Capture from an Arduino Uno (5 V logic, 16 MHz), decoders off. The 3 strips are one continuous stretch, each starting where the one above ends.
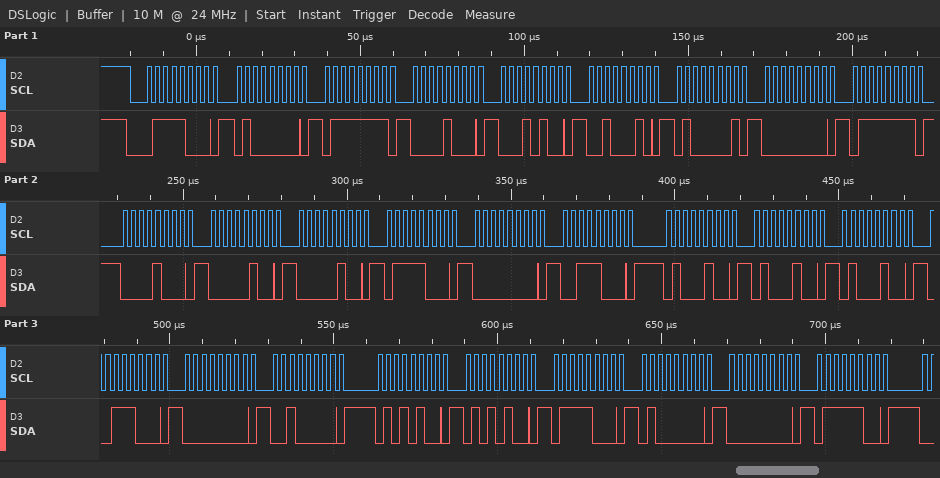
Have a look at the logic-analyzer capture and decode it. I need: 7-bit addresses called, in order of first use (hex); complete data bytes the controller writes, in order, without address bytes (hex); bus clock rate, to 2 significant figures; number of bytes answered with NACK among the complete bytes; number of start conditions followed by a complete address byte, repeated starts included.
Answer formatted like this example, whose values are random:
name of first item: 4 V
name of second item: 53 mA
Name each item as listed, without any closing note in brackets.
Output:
7-bit addresses called, in order of first use: 0x3C
complete data bytes the controller writes, in order, without address bytes: 40 7F 08 14 22 41 00 7F 08 04 04 78 00 38 44 44 44 38 00 20 54 54 78 40 00 7C
bus clock rate, to 2 significant figures: 400 kHz
number of bytes answered with NACK among the complete bytes: 0
number of start conditions followed by a complete address byte, repeated starts included: 1
